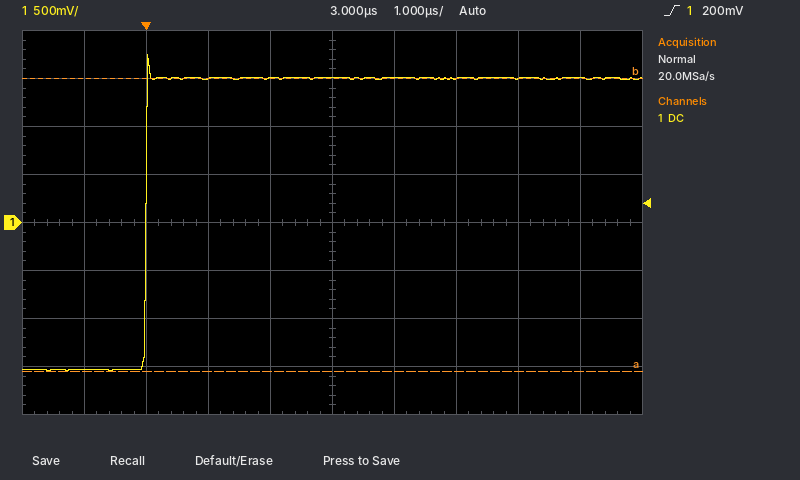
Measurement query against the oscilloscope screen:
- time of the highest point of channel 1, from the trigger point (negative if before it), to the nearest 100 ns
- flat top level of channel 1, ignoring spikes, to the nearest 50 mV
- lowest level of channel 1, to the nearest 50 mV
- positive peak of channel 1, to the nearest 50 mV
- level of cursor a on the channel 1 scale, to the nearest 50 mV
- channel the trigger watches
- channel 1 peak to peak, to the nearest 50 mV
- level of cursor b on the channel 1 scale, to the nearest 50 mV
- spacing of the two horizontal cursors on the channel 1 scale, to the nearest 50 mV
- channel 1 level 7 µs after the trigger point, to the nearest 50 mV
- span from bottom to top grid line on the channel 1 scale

0.0 µs
1.50 V
-1.55 V
1.75 V
-1.55 V
channel 1
3.30 V
1.50 V
3.05 V
1.50 V
4 V
